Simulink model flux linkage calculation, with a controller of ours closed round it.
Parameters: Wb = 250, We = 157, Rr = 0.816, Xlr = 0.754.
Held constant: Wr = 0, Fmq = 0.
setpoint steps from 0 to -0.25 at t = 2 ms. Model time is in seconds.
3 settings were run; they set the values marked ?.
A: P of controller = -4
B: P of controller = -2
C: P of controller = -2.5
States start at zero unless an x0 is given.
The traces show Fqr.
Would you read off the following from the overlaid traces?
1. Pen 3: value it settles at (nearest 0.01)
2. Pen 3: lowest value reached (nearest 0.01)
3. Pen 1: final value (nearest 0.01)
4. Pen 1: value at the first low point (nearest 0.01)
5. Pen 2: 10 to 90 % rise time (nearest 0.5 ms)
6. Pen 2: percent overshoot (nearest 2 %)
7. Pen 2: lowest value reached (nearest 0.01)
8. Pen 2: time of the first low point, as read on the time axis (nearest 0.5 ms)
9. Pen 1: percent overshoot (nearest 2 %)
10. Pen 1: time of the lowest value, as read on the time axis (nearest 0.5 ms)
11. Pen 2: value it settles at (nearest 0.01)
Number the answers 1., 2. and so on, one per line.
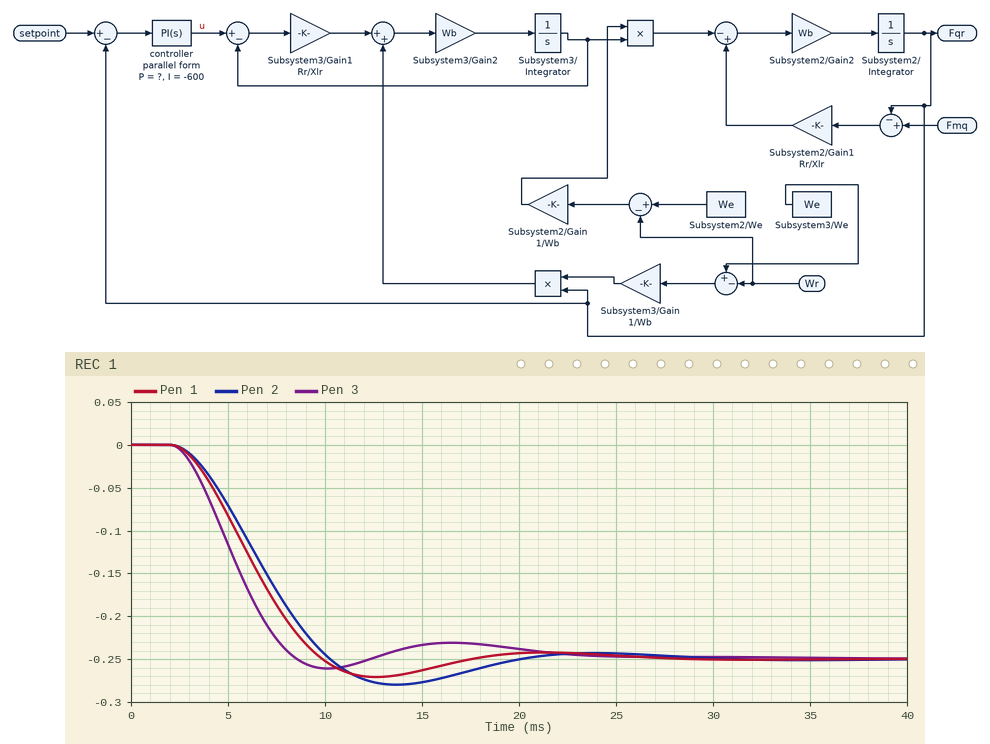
1. -0.25
2. -0.26
3. -0.25
4. -0.27
5. 5.5 ms
6. 12 %
7. -0.28
8. 13.5 ms
9. 8 %
10. 12.5 ms
11. -0.25
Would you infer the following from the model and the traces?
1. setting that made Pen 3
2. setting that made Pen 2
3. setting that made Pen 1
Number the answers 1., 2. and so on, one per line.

1. A
2. B
3. C
